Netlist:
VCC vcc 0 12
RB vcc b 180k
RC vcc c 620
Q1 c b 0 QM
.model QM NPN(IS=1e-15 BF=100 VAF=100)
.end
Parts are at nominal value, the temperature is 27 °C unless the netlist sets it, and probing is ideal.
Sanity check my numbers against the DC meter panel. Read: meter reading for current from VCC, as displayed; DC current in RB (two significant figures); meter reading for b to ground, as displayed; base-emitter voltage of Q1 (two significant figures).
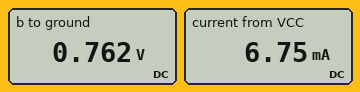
6.75 mA
62 µA
0.762 V
760 mV
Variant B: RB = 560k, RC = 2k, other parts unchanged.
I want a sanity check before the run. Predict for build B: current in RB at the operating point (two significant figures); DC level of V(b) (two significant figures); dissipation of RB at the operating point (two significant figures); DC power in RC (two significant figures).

20 µA
730 mV
230 µW
9.3 mW
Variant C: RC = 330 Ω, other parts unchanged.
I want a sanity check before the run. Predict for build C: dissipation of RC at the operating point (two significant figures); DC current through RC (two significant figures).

15 mW
6.8 mA
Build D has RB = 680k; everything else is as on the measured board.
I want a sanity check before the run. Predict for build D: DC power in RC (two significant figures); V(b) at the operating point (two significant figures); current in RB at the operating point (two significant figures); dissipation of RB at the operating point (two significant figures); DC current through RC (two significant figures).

2.1 mW
730 mV
17 µA
190 µW
1.8 mA
